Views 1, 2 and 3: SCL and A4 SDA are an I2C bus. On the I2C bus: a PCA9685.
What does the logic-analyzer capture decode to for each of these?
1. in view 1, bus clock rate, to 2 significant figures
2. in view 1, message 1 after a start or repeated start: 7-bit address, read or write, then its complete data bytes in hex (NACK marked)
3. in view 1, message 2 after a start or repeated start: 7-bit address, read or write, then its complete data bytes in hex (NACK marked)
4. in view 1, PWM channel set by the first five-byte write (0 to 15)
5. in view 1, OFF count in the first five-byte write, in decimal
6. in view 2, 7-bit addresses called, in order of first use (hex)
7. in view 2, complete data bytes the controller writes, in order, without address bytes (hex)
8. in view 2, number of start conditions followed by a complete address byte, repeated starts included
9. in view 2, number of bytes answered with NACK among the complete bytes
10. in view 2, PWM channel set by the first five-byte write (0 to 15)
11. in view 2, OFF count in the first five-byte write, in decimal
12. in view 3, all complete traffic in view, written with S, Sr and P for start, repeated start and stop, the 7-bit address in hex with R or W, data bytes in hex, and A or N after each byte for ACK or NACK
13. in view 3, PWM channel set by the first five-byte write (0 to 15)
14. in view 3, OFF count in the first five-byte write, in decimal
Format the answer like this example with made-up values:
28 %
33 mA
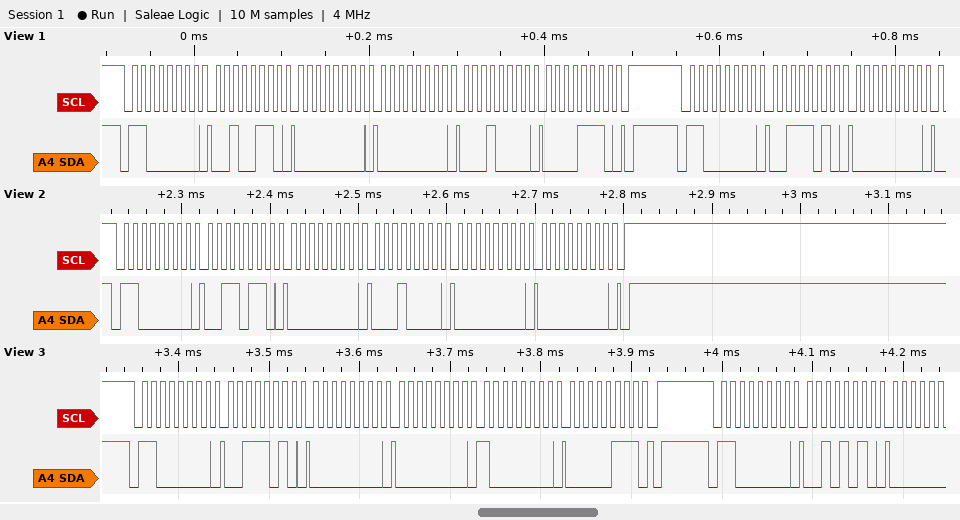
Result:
100 kHz
0x60 write: 26 00 00 10 0E
0x60 write: 3A 00
8
3600
0x60
36 00 10 00 00
1
0
12
0
S 60W A 3A A 00 A 00 A 80 A 07 A P S 60W A 2A A
13
1920
